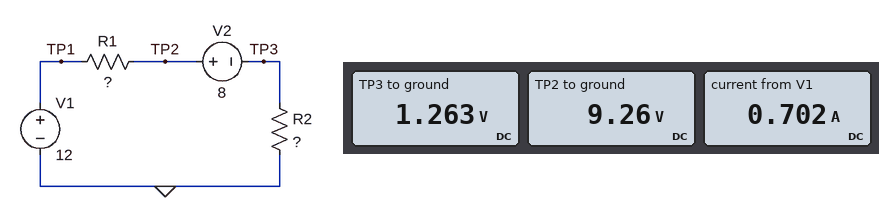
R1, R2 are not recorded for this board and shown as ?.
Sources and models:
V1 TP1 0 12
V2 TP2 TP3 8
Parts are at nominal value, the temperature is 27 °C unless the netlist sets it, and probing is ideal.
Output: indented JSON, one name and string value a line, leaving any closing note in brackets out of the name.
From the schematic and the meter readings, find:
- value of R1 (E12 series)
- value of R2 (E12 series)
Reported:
{
  "value of R1": "3.9 Ω",
  "value of R2": "1.8 Ω"
}
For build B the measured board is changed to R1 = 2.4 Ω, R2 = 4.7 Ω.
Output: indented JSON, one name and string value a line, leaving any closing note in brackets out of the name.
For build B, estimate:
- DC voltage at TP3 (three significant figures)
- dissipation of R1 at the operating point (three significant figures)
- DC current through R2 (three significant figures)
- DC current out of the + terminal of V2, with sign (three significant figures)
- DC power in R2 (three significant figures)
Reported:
{
  "DC voltage at TP3": "2.65 V",
  "dissipation of R1 at the operating point": "762 mW",
  "DC current through R2": "563 mA",
  "DC current out of the + terminal of V2, with sign": "-563 mA",
  "DC power in R2": "1.49 W"
}
